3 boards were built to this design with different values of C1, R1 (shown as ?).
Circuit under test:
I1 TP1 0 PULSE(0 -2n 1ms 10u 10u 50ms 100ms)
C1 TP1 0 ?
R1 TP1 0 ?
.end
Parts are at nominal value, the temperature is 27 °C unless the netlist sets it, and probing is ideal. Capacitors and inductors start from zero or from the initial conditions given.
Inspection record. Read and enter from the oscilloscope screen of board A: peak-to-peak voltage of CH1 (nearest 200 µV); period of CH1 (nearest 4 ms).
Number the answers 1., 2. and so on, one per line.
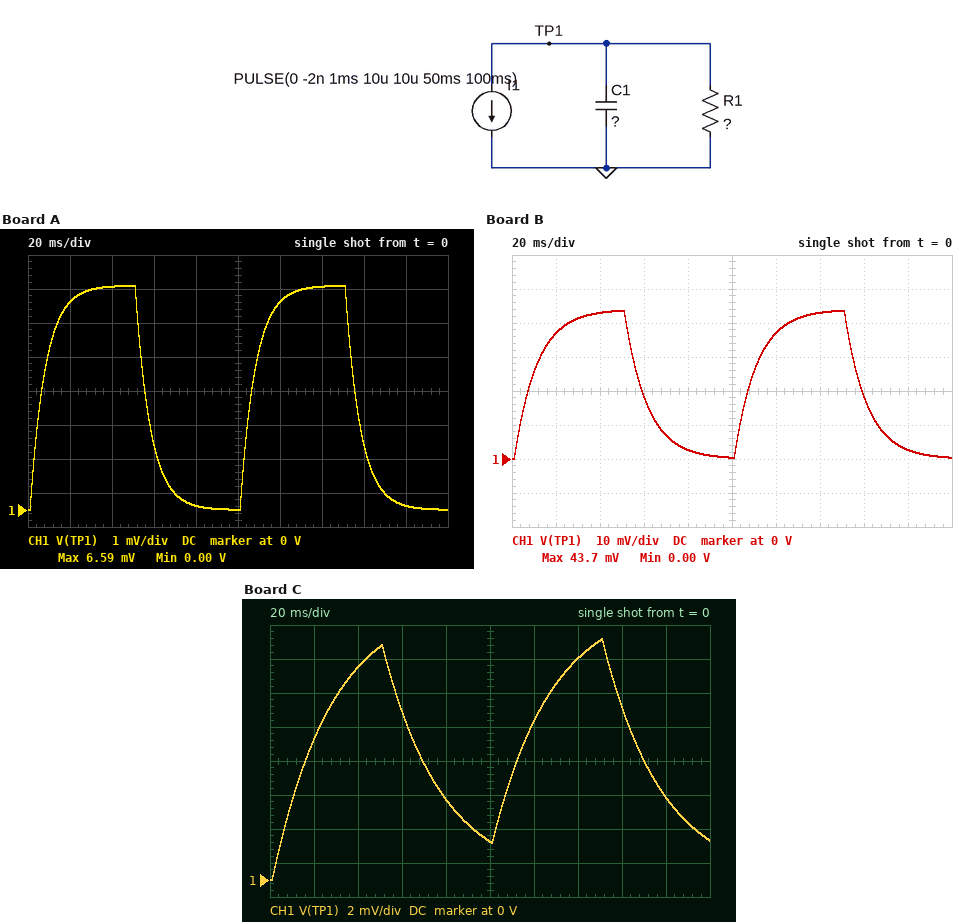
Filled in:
1. 6.6 mV
2. 100 ms
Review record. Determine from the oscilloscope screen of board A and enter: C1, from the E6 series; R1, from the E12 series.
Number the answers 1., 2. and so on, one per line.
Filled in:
1. 2.2 nF
2. 3.3 MΩ
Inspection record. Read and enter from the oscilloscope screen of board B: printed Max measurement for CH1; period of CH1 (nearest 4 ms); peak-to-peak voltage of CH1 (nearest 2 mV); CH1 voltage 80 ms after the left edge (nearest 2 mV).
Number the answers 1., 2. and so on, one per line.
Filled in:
1. 43.7 mV
2. 100 ms
3. 44 mV
4. 2 mV
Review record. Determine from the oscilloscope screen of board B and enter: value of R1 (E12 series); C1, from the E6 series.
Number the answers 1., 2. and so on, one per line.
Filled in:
1. 22 MΩ
2. 470 pF
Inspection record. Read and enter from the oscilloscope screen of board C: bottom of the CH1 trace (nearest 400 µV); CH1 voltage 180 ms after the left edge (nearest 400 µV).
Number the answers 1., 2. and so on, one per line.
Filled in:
1. 0 V
2. 4.8 mV
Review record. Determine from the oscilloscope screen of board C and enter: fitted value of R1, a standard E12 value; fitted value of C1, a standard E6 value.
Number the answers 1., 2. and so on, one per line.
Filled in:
1. 8.2 MΩ
2. 3.3 nF
